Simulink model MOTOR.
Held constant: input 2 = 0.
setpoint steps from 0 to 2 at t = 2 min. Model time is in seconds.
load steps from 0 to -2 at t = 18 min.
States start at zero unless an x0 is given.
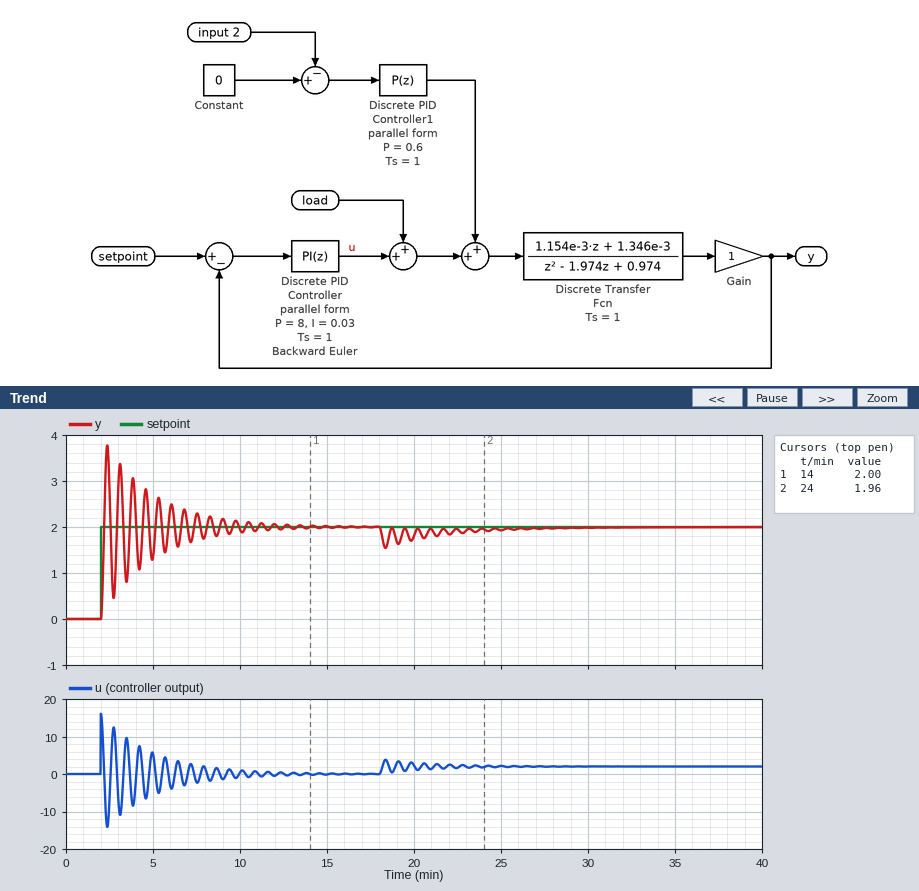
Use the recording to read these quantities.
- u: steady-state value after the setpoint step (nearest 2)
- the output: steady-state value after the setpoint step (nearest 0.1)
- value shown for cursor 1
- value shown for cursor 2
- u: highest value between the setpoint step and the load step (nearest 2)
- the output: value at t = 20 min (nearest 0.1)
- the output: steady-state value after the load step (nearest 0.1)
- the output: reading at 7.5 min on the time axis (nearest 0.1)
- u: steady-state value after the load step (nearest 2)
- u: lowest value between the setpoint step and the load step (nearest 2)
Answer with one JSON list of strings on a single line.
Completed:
["0", "2.0", "2.00", "1.96", "16", "1.8", "2.0", "2.3", "2", "-14"]
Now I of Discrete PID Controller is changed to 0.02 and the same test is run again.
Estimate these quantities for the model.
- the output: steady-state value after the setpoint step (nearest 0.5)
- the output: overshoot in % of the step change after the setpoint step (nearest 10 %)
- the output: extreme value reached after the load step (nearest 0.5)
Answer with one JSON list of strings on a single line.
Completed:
["2.0", "90 %", "1.5"]
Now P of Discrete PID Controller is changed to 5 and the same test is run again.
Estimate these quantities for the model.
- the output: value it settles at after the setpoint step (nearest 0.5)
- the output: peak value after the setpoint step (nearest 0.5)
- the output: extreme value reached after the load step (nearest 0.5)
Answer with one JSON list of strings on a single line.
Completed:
["2.0", "3.5", "1.5"]
